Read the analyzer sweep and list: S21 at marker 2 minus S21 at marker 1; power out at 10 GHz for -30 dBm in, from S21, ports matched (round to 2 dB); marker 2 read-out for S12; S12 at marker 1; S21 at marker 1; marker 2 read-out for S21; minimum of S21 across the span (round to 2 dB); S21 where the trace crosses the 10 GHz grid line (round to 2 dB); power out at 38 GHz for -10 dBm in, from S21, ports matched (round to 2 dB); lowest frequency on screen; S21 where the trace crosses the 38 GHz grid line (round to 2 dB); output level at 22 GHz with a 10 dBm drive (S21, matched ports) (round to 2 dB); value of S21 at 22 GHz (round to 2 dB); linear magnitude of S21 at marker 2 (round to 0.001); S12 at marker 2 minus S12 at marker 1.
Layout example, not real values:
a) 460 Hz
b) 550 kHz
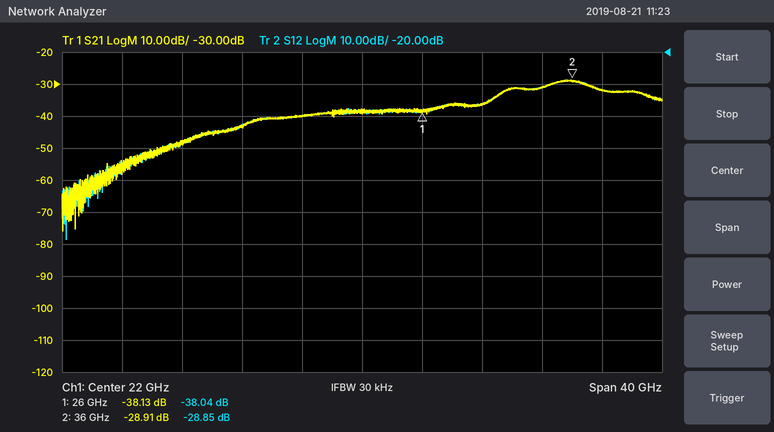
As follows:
a) 9.22 dB
b) -78 dBm
c) -28.85 dB
d) -38.04 dB
e) -38.13 dB
f) -28.91 dB
g) -76 dB
h) -48 dB
i) -42 dBm
j) 2 GHz
k) -32 dB
l) -28 dBm
m) -38 dB
n) 0.036
o) 9.19 dB
